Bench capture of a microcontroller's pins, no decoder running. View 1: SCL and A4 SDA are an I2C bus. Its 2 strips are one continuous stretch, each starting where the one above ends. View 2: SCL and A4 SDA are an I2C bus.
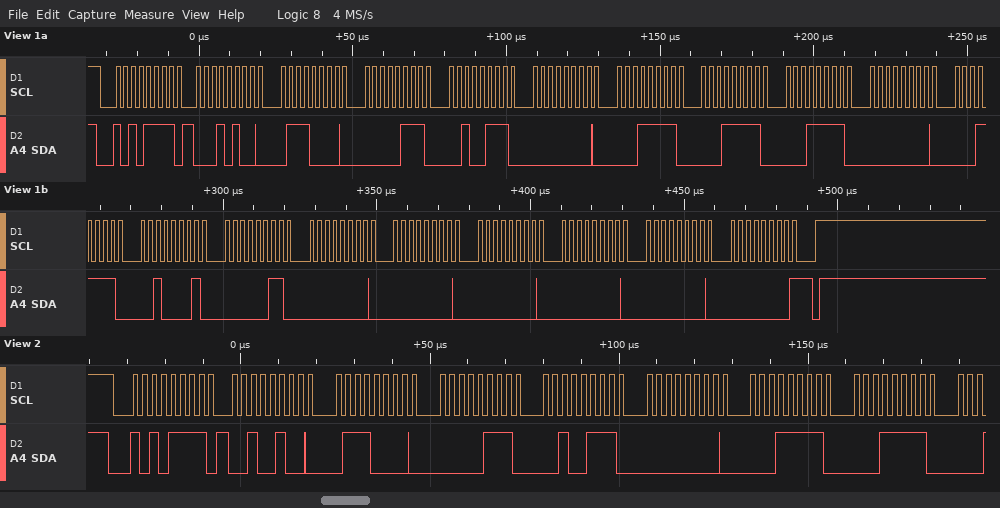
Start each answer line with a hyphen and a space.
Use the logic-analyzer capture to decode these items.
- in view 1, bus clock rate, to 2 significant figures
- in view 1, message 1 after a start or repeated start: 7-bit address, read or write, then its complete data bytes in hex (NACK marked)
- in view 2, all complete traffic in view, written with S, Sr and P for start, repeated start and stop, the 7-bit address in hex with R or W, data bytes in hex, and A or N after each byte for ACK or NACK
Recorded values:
- 400 kHz
- 0x57 read: 14 70 07 27 00 1F 1F 1F 00 1F 21 03 00 00 00 00 00 00 NACK
- S 57R A 24 A 70 A 07 A 27 A 00 A 1F A 1F A
